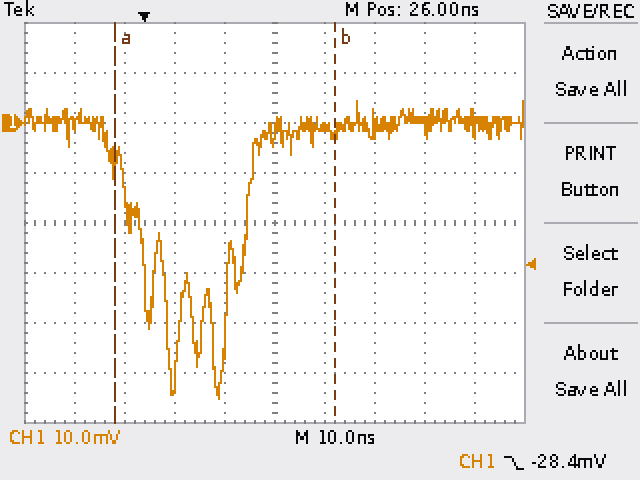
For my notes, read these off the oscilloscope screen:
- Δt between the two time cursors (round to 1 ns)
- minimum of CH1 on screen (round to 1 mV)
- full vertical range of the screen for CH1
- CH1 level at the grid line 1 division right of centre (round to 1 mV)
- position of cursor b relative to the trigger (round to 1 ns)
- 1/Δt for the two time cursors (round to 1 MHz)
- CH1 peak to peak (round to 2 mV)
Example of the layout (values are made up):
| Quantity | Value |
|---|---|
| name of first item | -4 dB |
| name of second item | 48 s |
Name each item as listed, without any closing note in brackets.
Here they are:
| Quantity | Value |
|---|---|
| Δt between the two time cursors | 44 ns |
| minimum of CH1 on screen | -55 mV |
| full vertical range of the screen for CH1 | 80 mV |
| CH1 level at the grid line 1 division right of centre | -1 mV |
| position of cursor b relative to the trigger | +38 ns |
| 1/Δt for the two time cursors | 23 MHz |
| CH1 peak to peak | 60 mV |
